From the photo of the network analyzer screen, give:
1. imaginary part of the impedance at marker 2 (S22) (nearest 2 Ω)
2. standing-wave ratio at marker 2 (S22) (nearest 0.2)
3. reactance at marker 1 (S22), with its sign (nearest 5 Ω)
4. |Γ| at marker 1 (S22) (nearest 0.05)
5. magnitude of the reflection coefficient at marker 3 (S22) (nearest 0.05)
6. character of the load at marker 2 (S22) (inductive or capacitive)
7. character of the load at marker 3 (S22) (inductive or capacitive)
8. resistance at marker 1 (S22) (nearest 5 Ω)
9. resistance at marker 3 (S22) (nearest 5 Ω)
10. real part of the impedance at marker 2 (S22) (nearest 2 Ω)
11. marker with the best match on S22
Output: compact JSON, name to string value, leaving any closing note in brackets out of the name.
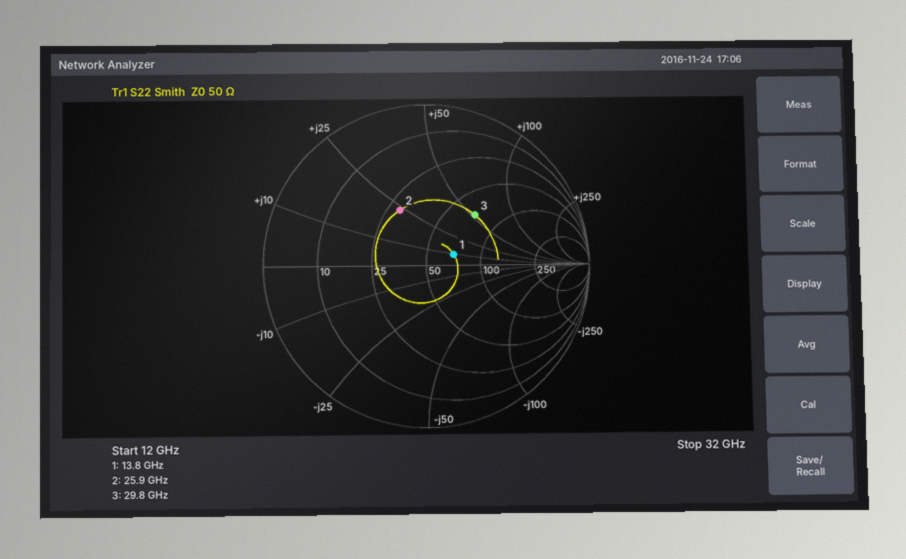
{"imaginary part of the impedance at marker 2 (S22)": "+24 Ω", "standing-wave ratio at marker 2 (S22)": "2.2", "reactance at marker 1 (S22), with its sign": "+10 Ω", "|Γ| at marker 1 (S22)": "0.20", "magnitude of the reflection coefficient at marker 3 (S22)": "0.45", "character of the load at marker 2 (S22)": "inductive", "character of the load at marker 3 (S22)": "inductive", "resistance at marker 1 (S22)": "70 Ω", "resistance at marker 3 (S22)": "70 Ω", "real part of the impedance at marker 2 (S22)": "30 Ω", "marker with the best match on S22": "marker 1"}
